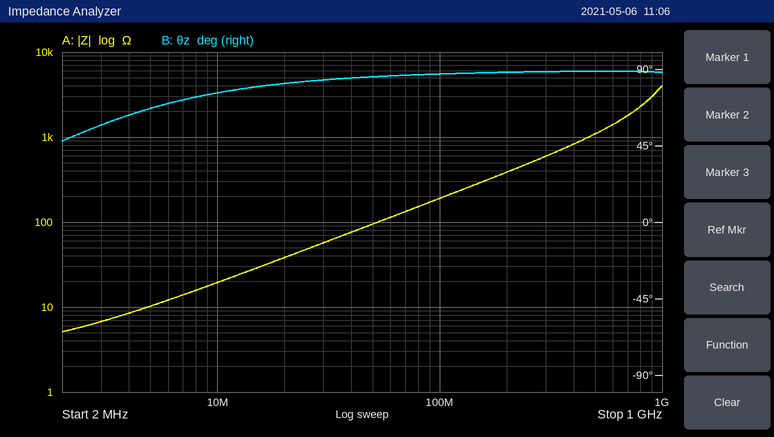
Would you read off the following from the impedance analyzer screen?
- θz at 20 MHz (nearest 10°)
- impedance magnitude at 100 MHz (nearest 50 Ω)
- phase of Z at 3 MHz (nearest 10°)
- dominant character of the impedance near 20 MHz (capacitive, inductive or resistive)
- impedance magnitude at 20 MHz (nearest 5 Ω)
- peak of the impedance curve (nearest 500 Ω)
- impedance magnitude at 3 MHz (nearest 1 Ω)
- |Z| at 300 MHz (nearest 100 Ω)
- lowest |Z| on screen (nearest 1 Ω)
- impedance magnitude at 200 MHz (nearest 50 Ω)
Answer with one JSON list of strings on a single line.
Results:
["80°", "200 Ω", "60°", "inductive", "40 Ω", "4.0 kΩ", "7 Ω", "600 Ω", "5 Ω", "400 Ω"]
